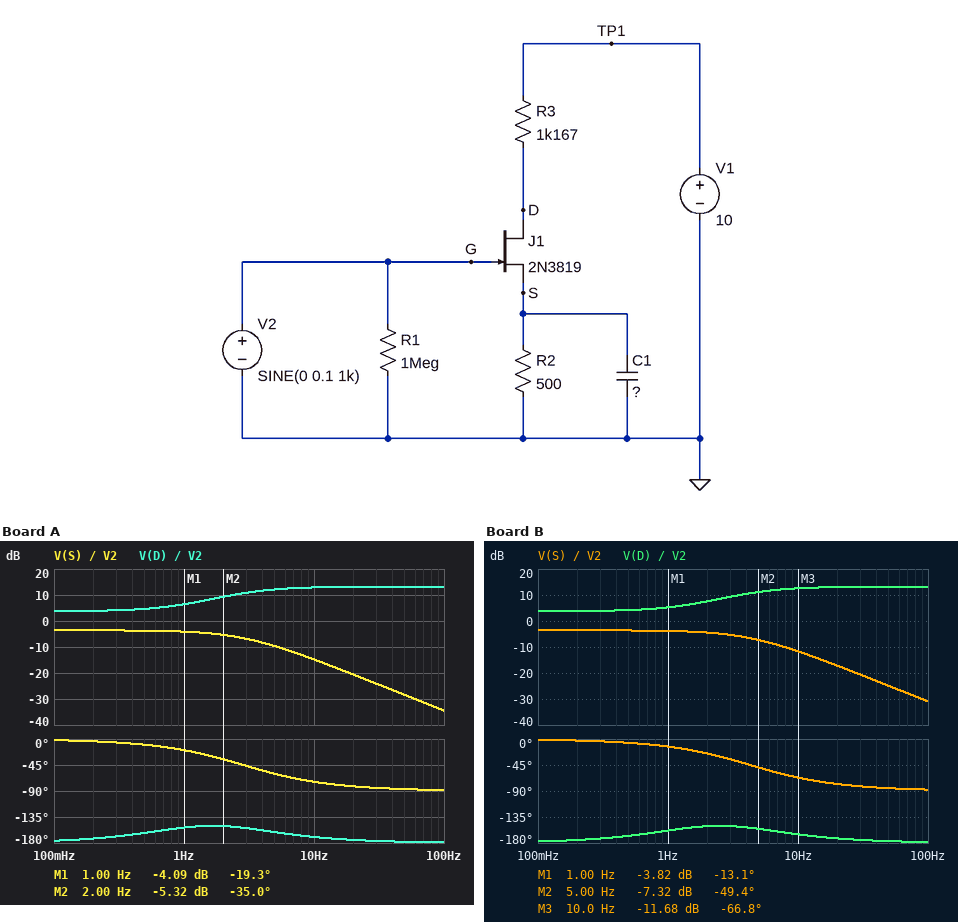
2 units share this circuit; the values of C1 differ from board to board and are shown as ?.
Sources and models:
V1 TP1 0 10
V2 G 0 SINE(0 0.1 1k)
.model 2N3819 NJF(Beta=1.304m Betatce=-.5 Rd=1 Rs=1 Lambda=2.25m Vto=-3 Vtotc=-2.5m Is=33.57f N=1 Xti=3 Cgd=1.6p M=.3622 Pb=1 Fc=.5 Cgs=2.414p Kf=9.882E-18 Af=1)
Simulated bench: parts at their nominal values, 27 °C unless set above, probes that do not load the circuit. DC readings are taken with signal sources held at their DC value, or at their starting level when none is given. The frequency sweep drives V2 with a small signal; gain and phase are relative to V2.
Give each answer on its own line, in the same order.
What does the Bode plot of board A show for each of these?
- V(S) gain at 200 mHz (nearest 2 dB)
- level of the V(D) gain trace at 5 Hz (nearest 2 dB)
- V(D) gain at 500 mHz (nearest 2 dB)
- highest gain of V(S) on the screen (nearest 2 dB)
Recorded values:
-4 dB
12 dB
4 dB
-4 dB
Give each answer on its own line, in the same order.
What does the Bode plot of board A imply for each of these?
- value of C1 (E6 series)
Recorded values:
330 µF
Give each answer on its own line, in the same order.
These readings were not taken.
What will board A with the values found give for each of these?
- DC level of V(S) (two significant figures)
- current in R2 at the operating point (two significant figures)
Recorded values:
1.5 V
3.0 mA
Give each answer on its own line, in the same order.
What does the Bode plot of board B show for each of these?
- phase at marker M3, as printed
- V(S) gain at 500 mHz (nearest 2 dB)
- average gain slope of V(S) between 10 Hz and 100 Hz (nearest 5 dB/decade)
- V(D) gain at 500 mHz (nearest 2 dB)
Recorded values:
-66.8 deg
-4 dB
-20 dB/decade
4 dB
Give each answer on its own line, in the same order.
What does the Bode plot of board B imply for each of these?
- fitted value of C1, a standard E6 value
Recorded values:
220 µF
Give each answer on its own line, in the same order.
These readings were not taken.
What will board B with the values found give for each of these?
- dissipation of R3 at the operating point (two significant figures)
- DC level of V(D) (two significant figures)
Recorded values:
10 mW
6.5 V
